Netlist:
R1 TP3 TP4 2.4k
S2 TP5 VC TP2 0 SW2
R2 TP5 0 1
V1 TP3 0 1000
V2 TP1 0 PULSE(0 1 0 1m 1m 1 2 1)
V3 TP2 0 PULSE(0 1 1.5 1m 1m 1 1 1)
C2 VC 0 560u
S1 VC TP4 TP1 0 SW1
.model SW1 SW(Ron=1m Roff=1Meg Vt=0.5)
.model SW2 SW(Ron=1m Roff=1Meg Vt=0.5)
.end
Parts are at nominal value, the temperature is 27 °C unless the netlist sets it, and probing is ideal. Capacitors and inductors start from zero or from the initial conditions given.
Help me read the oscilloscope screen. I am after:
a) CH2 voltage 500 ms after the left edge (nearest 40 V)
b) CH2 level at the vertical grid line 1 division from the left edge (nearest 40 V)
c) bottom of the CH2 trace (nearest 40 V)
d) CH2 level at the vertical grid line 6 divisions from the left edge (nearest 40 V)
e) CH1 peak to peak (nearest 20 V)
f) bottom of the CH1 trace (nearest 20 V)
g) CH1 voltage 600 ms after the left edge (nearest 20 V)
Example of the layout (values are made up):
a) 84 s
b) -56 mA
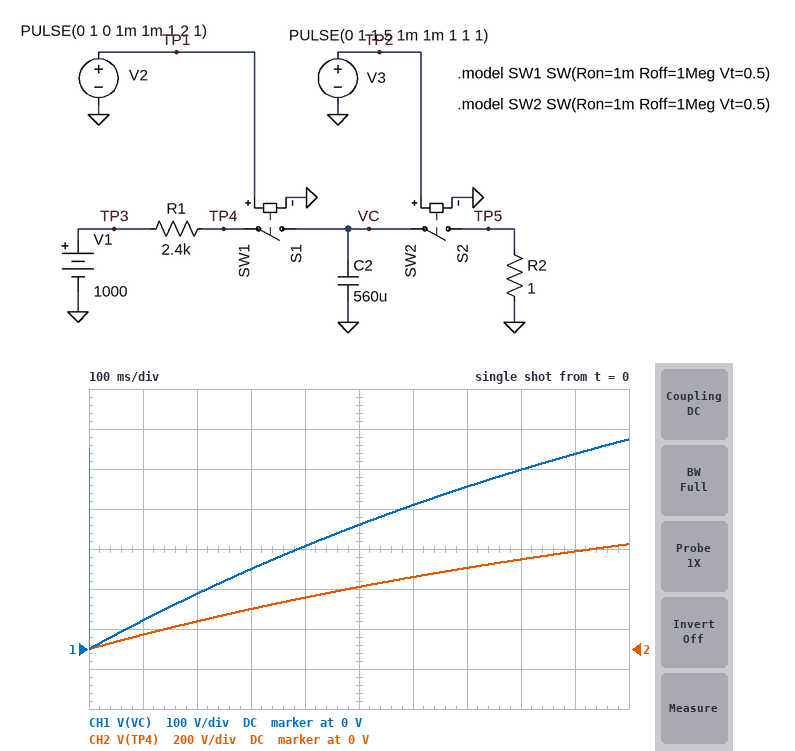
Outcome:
a) 320 V
b) 80 V
c) 0 V
d) 360 V
e) 520 V
f) 0 V
g) 360 V
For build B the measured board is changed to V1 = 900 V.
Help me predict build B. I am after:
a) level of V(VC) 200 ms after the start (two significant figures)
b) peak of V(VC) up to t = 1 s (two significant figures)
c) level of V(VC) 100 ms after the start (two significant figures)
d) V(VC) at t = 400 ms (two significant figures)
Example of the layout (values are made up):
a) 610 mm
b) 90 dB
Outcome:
a) 120 V
b) 470 V
c) 64 V
d) 230 V
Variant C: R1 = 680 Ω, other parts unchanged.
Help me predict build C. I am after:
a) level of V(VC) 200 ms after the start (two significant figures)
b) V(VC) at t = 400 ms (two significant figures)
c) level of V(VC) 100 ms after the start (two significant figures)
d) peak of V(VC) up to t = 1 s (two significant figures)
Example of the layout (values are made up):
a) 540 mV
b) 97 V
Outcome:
a) 410 V
b) 650 V
c) 230 V
d) 930 V
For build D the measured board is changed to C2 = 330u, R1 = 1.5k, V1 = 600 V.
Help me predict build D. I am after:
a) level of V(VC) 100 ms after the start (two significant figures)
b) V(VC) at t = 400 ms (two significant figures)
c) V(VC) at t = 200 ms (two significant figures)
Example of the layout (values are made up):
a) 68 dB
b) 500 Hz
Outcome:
a) 110 V
b) 330 V
c) 200 V
